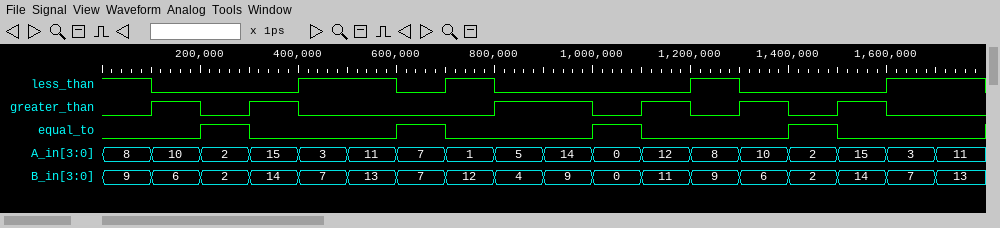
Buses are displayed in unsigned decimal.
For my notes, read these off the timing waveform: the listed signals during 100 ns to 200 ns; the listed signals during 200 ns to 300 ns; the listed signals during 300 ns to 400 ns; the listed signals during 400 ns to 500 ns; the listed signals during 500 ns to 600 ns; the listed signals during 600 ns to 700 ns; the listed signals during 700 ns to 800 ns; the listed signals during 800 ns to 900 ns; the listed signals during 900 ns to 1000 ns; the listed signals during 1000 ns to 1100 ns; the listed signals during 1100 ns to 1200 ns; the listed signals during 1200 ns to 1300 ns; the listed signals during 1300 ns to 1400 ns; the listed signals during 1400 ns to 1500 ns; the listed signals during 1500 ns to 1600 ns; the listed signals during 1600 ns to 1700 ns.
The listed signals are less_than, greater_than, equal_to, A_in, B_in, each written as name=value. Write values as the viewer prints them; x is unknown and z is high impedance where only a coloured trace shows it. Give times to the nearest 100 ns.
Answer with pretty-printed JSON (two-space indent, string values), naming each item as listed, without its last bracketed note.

{
  "the listed signals during 100 ns to 200 ns": "less_than=0, greater_than=1, equal_to=0, A_in=10, B_in=6",
  "the listed signals during 200 ns to 300 ns": "less_than=0, greater_than=0, equal_to=1, A_in=2, B_in=2",
  "the listed signals during 300 ns to 400 ns": "less_than=0, greater_than=1, equal_to=0, A_in=15, B_in=14",
  "the listed signals during 400 ns to 500 ns": "less_than=1, greater_than=0, equal_to=0, A_in=3, B_in=7",
  "the listed signals during 500 ns to 600 ns": "less_than=1, greater_than=0, equal_to=0, A_in=11, B_in=13",
  "the listed signals during 600 ns to 700 ns": "less_than=0, greater_than=0, equal_to=1, A_in=7, B_in=7",
  "the listed signals during 700 ns to 800 ns": "less_than=1, greater_than=0, equal_to=0, A_in=1, B_in=12",
  "the listed signals during 800 ns to 900 ns": "less_than=0, greater_than=1, equal_to=0, A_in=5, B_in=4",
  "the listed signals during 900 ns to 1000 ns": "less_than=0, greater_than=1, equal_to=0, A_in=14, B_in=9",
  "the listed signals during 1000 ns to 1100 ns": "less_than=0, greater_than=0, equal_to=1, A_in=0, B_in=0",
  "the listed signals during 1100 ns to 1200 ns": "less_than=0, greater_than=1, equal_to=0, A_in=12, B_in=11",
  "the listed signals during 1200 ns to 1300 ns": "less_than=1, greater_than=0, equal_to=0, A_in=8, B_in=9",
  "the listed signals during 1300 ns to 1400 ns": "less_than=0, greater_than=1, equal_to=0, A_in=10, B_in=6",
  "the listed signals during 1400 ns to 1500 ns": "less_than=0, greater_than=0, equal_to=1, A_in=2, B_in=2",
  "the listed signals during 1500 ns to 1600 ns": "less_than=0, greater_than=1, equal_to=0, A_in=15, B_in=14",
  "the listed signals during 1600 ns to 1700 ns": "less_than=1, greater_than=0, equal_to=0, A_in=3, B_in=7"
}
